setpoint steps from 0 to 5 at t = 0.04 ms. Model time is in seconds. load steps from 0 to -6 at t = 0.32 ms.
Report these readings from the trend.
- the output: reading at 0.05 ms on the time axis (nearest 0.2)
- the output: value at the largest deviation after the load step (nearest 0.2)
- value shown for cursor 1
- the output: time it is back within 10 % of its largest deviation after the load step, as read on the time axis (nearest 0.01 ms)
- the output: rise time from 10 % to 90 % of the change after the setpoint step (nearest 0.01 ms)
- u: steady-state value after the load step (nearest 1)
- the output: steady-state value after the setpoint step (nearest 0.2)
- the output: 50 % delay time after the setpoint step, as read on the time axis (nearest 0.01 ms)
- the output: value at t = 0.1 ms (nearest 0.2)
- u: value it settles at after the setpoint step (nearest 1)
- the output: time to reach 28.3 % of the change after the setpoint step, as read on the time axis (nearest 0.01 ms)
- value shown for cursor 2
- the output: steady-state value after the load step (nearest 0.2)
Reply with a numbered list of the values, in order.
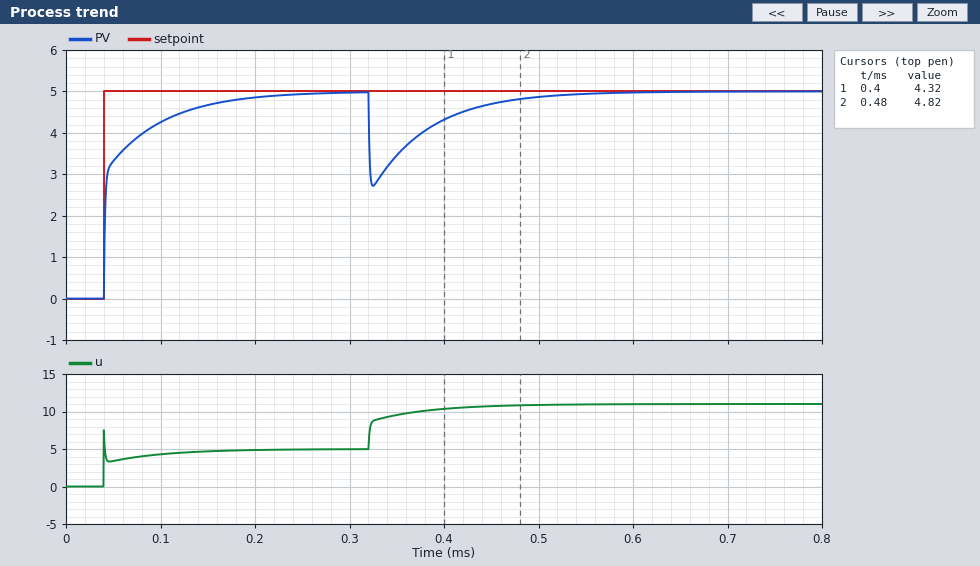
1. 3.4
2. 2.8
3. 4.32
4. 0.47 ms
5. 0.08 ms
6. 11
7. 5.0
8. 0.04 ms
9. 4.2
10. 5
11. 0.04 ms
12. 4.82
13. 5.0
